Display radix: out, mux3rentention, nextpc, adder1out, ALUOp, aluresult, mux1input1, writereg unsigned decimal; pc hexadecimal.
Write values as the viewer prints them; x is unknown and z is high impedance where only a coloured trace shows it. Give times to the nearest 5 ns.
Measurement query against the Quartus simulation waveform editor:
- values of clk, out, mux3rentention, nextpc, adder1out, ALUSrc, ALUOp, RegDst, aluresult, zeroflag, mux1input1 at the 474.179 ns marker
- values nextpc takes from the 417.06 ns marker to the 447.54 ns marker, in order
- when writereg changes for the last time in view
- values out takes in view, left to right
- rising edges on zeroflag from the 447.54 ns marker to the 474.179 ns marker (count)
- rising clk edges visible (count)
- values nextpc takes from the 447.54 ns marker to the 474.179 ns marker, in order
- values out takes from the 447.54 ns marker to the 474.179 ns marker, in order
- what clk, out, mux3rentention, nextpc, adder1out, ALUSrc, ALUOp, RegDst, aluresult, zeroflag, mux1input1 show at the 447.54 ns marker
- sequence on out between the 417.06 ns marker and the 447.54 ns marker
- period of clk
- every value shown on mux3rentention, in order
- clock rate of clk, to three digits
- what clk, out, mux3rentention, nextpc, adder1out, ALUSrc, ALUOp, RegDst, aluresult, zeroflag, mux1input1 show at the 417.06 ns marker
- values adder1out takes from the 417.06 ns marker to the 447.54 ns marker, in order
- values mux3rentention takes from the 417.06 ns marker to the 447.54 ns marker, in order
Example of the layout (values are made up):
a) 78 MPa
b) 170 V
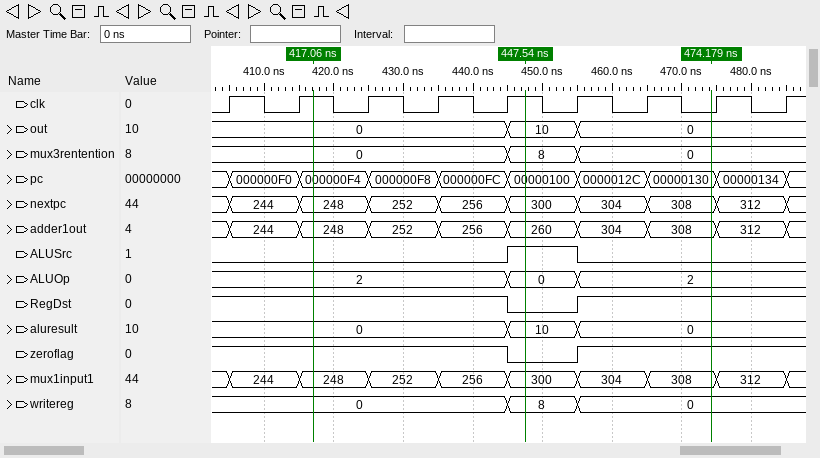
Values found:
a) clk=0, out=0, mux3rentention=0, nextpc=308, adder1out=308, ALUSrc=0, ALUOp=2, RegDst=1, aluresult=0, zeroflag=1, mux1input1=308
b) 248, 252, 256, 300
c) 455 ns
d) 0, 10, 0
e) 1
f) 9
g) 300, 304, 308
h) 10, 0
i) clk=1, out=10, mux3rentention=8, nextpc=300, adder1out=260, ALUSrc=1, ALUOp=0, RegDst=0, aluresult=10, zeroflag=0, mux1input1=300
j) 0, 10
k) 10 ns
l) 0, 8, 0
m) 100 MHz
n) clk=1, out=0, mux3rentention=0, nextpc=248, adder1out=248, ALUSrc=0, ALUOp=2, RegDst=1, aluresult=0, zeroflag=1, mux1input1=248
o) 248, 252, 256, 260
p) 0, 8
